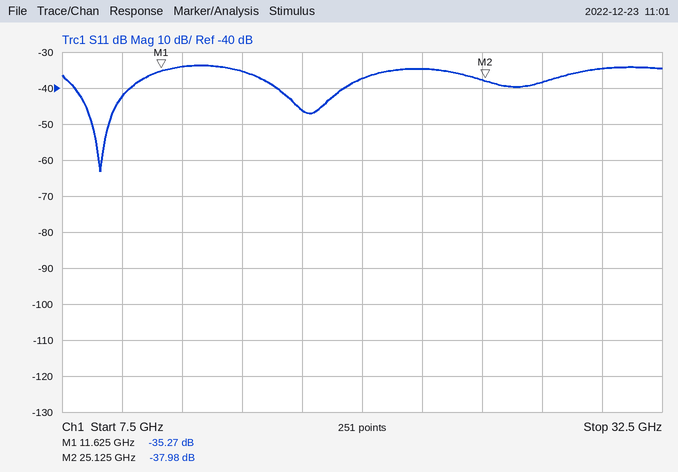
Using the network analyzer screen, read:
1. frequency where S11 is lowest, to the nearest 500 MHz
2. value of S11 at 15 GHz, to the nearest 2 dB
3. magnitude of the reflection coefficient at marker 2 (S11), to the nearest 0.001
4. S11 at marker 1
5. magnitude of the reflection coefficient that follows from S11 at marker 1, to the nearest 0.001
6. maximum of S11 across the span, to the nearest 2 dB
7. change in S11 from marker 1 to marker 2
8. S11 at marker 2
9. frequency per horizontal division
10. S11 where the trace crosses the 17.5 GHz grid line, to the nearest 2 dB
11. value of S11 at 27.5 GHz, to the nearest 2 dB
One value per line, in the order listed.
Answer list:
9.0 GHz
-36 dB
0.013
-35.27 dB
0.017
-34 dB
-2.71 dB
-37.98 dB
2.5 GHz
-46 dB
-38 dB
